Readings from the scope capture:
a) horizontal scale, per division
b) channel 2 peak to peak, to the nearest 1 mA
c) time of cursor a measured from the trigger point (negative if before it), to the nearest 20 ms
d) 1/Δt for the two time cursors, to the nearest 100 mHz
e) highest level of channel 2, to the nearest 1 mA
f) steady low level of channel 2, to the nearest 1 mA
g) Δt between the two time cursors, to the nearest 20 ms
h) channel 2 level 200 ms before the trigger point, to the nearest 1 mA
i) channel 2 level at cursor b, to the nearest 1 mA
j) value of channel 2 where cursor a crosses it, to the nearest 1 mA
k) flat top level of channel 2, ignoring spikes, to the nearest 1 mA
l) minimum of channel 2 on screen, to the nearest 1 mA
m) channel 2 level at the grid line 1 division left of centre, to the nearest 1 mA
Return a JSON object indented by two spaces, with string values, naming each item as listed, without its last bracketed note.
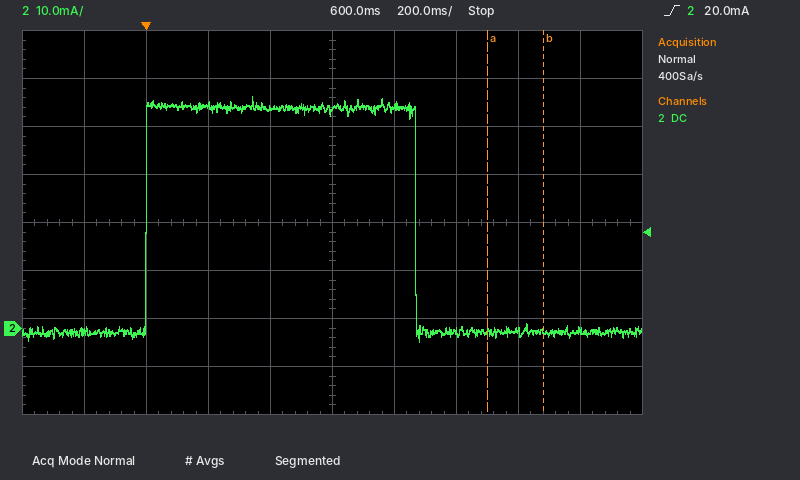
{
  "horizontal scale, per division": "200 ms",
  "channel 2 peak to peak, to the nearest 1 mA": "51 mA",
  "time of cursor a measured from the trigger point (negative if before it), to the nearest 20 ms": "+1.10 s",
  "1/Δt for the two time cursors, to the nearest 100 mHz": "5.6 Hz",
  "highest level of channel 2, to the nearest 1 mA": "48 mA",
  "steady low level of channel 2, to the nearest 1 mA": "-1 mA",
  "Δt between the two time cursors, to the nearest 20 ms": "180 ms",
  "channel 2 level 200 ms before the trigger point, to the nearest 1 mA": "-1 mA",
  "channel 2 level at cursor b, to the nearest 1 mA": "-1 mA",
  "value of channel 2 where cursor a crosses it, to the nearest 1 mA": "-1 mA",
  "flat top level of channel 2, ignoring spikes, to the nearest 1 mA": "46 mA",
  "minimum of channel 2 on screen, to the nearest 1 mA": "-3 mA",
  "channel 2 level at the grid line 1 division left of centre, to the nearest 1 mA": "46 mA"
}
